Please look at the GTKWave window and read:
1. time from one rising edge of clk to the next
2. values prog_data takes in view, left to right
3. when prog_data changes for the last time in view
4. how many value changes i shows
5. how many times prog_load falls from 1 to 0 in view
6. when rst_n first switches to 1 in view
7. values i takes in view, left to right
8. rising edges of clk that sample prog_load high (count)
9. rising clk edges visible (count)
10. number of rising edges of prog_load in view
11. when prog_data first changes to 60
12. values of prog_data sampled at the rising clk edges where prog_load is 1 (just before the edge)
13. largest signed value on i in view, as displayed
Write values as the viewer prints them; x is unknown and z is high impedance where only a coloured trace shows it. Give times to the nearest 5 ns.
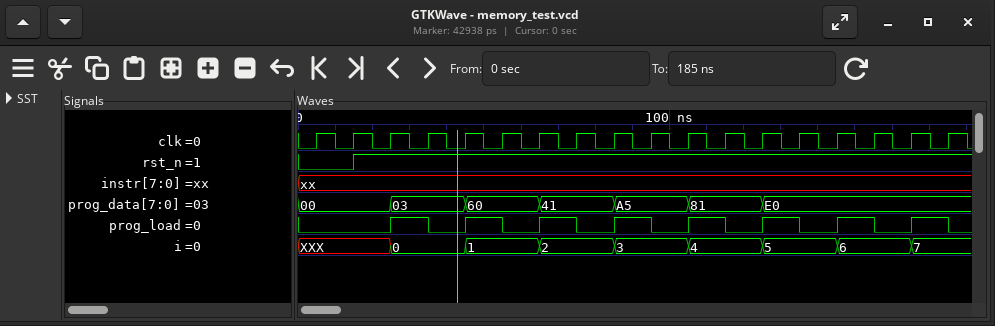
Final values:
10 ns
00, 03, 60, 41, A5, 81, E0
125 ns
8
8
15 ns
XXX, 0, 1, 2, 3, 4, 5, 6, 7
8
18
8
45 ns
03, 60, 41, A5, 81, E0, E0, E0
7
